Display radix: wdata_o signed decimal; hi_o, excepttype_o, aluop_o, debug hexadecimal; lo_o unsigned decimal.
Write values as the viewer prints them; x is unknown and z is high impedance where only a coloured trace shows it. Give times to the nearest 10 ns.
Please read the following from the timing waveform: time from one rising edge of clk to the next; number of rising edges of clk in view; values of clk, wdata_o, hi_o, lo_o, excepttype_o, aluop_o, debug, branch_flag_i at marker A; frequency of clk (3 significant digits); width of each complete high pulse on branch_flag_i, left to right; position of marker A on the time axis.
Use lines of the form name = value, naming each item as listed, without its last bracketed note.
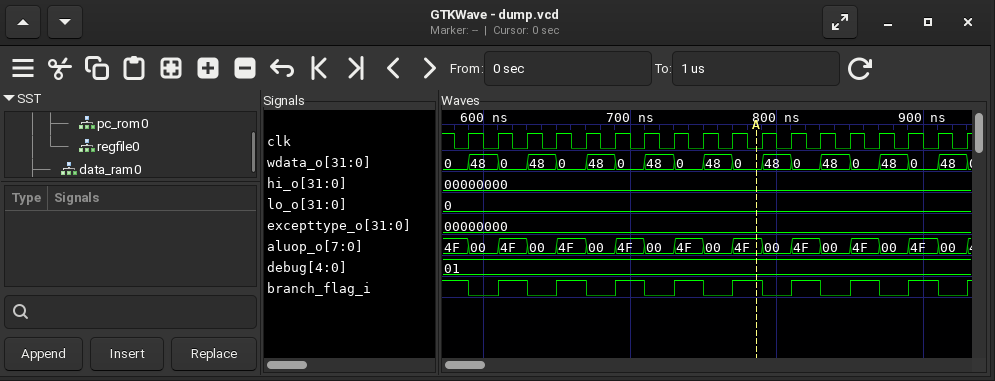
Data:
time from one rising edge of clk to the next = 20 ns
number of rising edges of clk in view = 18
values of clk, wdata_o, hi_o, lo_o, excepttype_o, aluop_o, debug, branch_flag_i at marker A = clk=0, wdata_o=0, hi_o=00000000, lo_o=0, excepttype_o=00000000, aluop_o=4F, debug=01, branch_flag_i=1
frequency of clk = 50.0 MHz
width of each complete high pulse on branch_flag_i, left to right = 20 ns, 20 ns, 20 ns, 20 ns, 20 ns, 20 ns, 20 ns, 20 ns
position of marker A on the time axis = 790 ns
